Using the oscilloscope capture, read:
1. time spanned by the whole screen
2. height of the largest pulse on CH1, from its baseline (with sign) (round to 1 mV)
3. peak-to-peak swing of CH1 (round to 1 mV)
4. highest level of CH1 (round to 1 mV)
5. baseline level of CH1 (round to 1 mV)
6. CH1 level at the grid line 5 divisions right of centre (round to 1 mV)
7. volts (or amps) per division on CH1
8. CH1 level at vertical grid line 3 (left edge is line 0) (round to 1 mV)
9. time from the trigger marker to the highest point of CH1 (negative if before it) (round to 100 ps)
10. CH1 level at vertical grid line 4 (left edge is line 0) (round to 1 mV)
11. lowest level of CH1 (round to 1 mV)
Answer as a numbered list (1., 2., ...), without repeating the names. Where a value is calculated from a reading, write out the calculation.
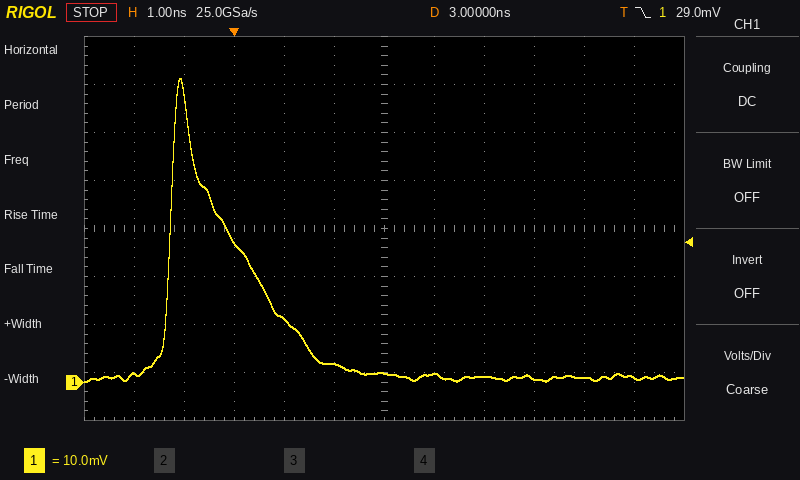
1. 12 ns
2. 63 mV − (1 mV) = +62 mV
3. 63 mV − (0 mV) = 63 mV
4. 63 mV
5. 1 mV
6. 1 mV
7. 10 mV
8. 29 mV
9. -1.1 ns
10. 13 mV
11. 0 mV
